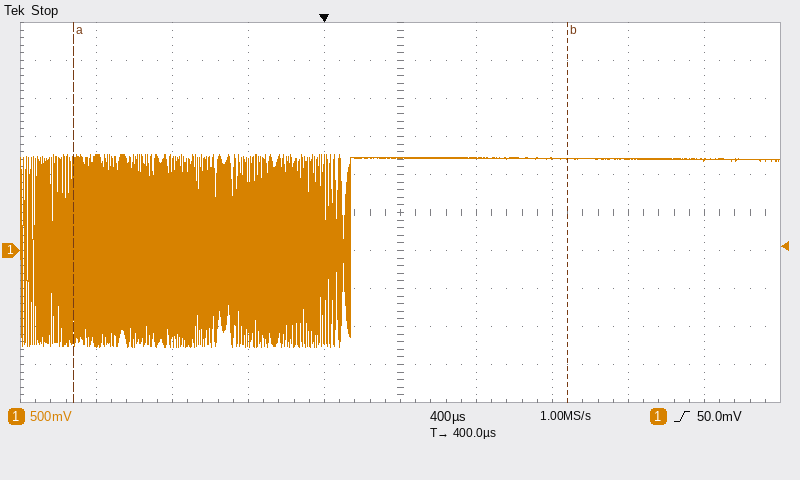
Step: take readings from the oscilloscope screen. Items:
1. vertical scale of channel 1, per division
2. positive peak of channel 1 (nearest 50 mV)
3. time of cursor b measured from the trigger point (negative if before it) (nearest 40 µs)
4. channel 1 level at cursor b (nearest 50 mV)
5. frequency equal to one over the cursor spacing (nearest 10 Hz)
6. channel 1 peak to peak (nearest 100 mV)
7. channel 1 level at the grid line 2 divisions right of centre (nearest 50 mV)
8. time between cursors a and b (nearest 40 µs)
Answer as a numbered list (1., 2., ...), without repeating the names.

1. 500 mV
2. 1.25 V
3. +1.28 ms
4. 1.20 V
5. 380 Hz
6. 2.50 V
7. 1.20 V
8. 2.60 ms
